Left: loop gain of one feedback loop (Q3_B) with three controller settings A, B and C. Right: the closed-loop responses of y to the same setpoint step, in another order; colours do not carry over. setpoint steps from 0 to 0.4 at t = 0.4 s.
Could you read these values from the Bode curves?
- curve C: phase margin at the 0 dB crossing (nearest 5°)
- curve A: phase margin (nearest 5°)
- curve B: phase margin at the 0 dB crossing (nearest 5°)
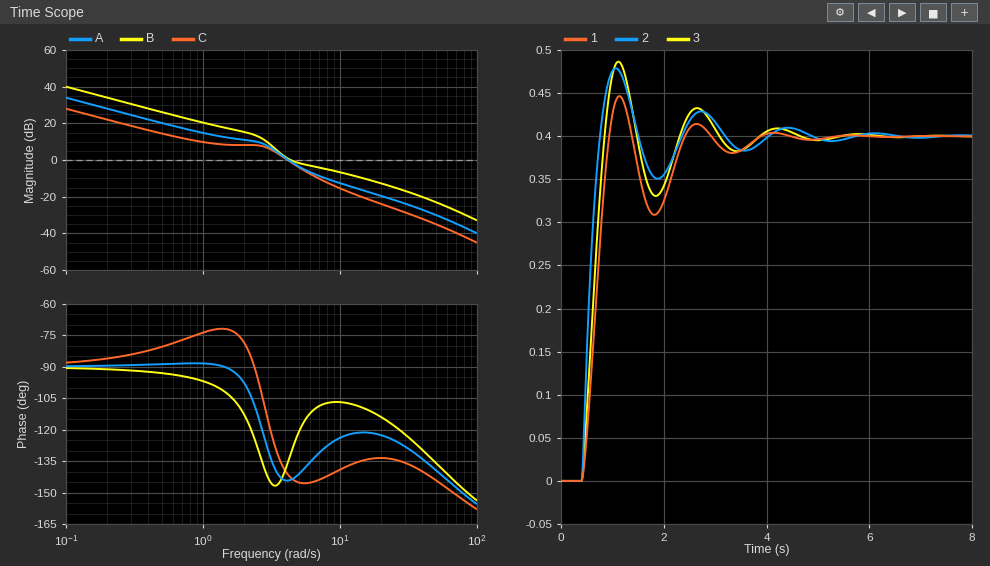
40°
35°
50°
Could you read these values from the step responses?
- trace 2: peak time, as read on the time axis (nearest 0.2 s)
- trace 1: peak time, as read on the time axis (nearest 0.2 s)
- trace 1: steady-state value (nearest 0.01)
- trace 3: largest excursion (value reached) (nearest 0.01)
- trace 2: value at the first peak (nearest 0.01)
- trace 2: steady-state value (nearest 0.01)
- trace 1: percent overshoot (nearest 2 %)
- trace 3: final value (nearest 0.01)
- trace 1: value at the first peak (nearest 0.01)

1.0 s
1.2 s
0.40
0.49
0.48
0.40
12 %
0.40
0.45
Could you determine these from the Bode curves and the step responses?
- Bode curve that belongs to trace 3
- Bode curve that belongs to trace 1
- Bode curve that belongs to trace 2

A
C
B
